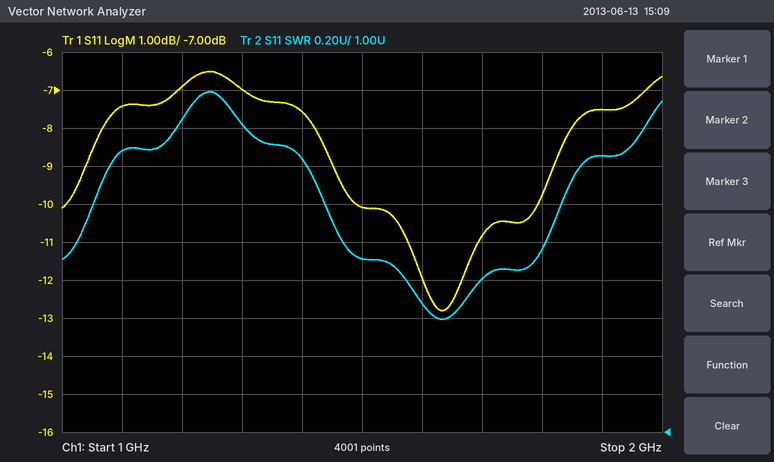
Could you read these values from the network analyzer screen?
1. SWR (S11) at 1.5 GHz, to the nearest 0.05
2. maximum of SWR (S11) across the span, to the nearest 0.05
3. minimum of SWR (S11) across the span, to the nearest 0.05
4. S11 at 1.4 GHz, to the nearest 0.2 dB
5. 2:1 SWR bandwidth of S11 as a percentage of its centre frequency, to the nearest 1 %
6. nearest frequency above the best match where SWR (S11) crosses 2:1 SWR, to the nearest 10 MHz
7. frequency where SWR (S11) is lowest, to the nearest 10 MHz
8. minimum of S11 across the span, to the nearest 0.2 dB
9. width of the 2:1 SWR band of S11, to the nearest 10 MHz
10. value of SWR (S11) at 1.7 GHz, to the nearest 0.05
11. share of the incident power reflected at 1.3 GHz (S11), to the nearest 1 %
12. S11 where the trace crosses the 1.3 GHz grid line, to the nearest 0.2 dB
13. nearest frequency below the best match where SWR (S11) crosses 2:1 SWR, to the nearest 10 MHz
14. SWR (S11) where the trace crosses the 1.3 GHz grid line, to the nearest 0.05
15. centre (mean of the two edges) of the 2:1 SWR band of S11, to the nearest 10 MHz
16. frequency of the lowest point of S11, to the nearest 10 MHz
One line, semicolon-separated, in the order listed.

1.90; 2.80; 1.60; -7.6 dB; 21 %; 1.81 GHz; 1.63 GHz; -12.8 dB; 340 MHz; 1.80; 20 %; -7.0 dB; 1.47 GHz; 2.60; 1.64 GHz; 1.63 GHz
